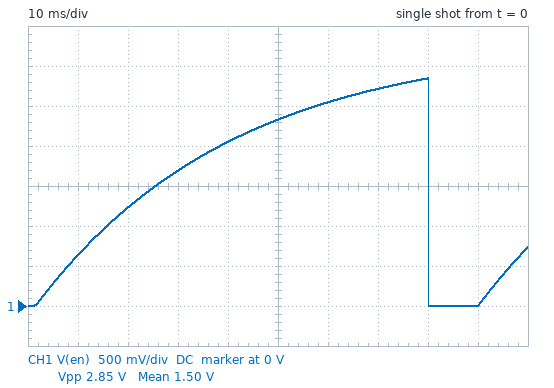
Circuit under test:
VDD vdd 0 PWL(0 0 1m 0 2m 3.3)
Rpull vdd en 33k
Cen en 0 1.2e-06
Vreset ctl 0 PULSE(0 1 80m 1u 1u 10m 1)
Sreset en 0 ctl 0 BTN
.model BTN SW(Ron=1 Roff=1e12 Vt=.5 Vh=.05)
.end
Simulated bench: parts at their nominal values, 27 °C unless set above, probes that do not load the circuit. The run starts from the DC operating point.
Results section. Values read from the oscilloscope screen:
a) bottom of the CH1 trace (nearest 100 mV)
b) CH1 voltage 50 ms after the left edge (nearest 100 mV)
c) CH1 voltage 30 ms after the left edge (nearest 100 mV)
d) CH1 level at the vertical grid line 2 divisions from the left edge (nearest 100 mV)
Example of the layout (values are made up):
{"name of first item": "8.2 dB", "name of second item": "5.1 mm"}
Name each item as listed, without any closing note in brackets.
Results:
{"bottom of the CH1 trace": "0 V", "CH1 voltage 50 ms after the left edge": "2.3 V", "CH1 voltage 30 ms after the left edge": "1.7 V", "CH1 level at the vertical grid line 2 divisions from the left edge": "1.2 V"}
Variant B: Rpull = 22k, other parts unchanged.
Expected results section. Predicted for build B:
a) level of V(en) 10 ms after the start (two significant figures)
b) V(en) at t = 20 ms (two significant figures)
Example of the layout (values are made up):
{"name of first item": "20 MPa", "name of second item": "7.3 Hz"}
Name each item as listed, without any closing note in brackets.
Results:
{"level of V(en) 10 ms after the start": "910 mV", "V(en) at t = 20 ms": "1.7 V"}
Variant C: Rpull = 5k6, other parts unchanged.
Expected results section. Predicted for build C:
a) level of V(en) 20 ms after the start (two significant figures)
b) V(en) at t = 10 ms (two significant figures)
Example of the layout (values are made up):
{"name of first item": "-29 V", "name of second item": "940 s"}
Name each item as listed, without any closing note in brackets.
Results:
{"level of V(en) 20 ms after the start": "3.1 V", "V(en) at t = 10 ms": "2.4 V"}
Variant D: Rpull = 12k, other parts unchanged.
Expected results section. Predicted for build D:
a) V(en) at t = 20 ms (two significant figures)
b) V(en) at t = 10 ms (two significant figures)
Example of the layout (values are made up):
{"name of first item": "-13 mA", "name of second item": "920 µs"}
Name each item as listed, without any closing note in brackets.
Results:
{"V(en) at t = 20 ms": "2.4 V", "V(en) at t = 10 ms": "1.5 V"}
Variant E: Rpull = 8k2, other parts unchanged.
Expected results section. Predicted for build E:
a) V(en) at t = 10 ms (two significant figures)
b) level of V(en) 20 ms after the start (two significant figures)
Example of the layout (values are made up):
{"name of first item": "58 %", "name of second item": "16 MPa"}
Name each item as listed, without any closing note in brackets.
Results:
{"V(en) at t = 10 ms": "1.9 V", "level of V(en) 20 ms after the start": "2.8 V"}
